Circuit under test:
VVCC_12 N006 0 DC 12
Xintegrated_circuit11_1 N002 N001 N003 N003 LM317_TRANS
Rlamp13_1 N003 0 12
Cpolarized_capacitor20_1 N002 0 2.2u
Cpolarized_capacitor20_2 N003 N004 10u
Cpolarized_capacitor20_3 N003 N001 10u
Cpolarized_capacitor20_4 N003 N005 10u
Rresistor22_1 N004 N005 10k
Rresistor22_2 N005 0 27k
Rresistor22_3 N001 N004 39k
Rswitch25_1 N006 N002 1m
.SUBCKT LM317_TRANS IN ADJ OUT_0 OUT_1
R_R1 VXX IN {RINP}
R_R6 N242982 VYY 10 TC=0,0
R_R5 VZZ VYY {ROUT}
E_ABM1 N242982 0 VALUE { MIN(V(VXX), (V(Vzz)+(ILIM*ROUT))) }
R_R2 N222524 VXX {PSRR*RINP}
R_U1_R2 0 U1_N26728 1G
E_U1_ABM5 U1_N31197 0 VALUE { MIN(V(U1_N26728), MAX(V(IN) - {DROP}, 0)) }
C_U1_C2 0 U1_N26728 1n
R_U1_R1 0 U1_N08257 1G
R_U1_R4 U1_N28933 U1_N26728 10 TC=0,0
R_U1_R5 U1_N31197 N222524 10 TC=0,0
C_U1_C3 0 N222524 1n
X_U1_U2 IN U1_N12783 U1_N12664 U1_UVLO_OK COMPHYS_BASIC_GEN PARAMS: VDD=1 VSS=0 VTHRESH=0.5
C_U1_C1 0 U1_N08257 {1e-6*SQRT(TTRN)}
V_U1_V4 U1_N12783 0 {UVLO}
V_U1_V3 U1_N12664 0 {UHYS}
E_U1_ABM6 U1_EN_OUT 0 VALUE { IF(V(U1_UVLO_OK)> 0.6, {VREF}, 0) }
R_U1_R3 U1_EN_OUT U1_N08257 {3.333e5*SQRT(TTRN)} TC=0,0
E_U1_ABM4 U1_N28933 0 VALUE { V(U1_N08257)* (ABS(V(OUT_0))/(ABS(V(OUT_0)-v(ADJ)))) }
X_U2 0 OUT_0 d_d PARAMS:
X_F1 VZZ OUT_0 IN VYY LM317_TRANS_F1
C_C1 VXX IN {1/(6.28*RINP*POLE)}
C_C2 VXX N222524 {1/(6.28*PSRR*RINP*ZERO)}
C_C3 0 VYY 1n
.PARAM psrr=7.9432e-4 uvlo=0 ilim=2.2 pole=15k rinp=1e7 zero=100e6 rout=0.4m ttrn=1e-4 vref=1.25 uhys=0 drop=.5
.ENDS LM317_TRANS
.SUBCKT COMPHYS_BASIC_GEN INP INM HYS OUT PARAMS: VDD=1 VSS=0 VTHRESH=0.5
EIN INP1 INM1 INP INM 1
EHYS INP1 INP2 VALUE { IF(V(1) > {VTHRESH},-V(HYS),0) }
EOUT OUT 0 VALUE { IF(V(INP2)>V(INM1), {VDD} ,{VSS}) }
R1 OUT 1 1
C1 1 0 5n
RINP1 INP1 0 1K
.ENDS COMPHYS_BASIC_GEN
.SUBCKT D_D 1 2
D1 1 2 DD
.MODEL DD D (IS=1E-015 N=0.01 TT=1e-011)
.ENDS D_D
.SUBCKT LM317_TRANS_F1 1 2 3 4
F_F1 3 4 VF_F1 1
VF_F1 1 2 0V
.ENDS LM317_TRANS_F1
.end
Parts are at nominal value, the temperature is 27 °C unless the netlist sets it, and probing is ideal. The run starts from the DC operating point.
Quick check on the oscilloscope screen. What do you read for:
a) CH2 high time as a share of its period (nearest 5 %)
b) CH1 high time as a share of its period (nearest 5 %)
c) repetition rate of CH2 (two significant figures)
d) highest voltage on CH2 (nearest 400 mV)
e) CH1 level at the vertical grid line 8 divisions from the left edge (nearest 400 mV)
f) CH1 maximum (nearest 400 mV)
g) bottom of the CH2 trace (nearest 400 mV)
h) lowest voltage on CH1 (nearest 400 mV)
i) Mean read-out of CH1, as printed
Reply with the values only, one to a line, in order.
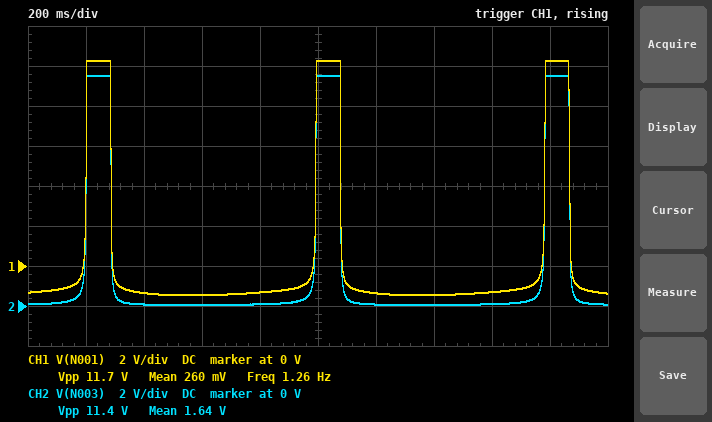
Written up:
10 %
10 %
1.3 Hz
11.6 V
-1.2 V
10.4 V
0 V
-1.6 V
260 mV
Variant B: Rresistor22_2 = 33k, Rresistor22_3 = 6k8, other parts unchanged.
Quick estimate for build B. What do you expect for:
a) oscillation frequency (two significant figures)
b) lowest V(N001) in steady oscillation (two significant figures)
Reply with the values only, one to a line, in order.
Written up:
2.6 Hz
-1.3 V
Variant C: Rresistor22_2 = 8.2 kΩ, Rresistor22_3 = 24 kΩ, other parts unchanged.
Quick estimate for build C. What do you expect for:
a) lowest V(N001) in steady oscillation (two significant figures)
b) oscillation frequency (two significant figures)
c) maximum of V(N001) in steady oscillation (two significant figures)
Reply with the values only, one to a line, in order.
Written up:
-1.6 V
2.1 Hz
10 V
